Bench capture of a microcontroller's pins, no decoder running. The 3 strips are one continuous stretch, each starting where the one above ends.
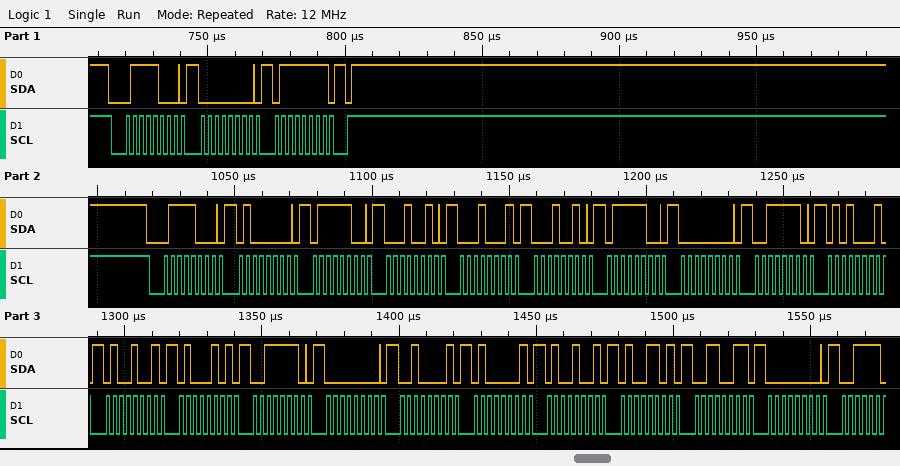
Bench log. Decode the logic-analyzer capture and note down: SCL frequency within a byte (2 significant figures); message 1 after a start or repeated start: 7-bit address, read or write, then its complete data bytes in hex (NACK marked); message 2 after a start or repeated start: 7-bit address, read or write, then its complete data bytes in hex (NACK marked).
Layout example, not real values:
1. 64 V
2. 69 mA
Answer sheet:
1. 400 kHz
2. 0x3C write: 00 7F
3. 0x3C write: 40 7C 12 11 12 7C 00 3E 51 49 45 3E 00 21 41 49 4D 33 00
